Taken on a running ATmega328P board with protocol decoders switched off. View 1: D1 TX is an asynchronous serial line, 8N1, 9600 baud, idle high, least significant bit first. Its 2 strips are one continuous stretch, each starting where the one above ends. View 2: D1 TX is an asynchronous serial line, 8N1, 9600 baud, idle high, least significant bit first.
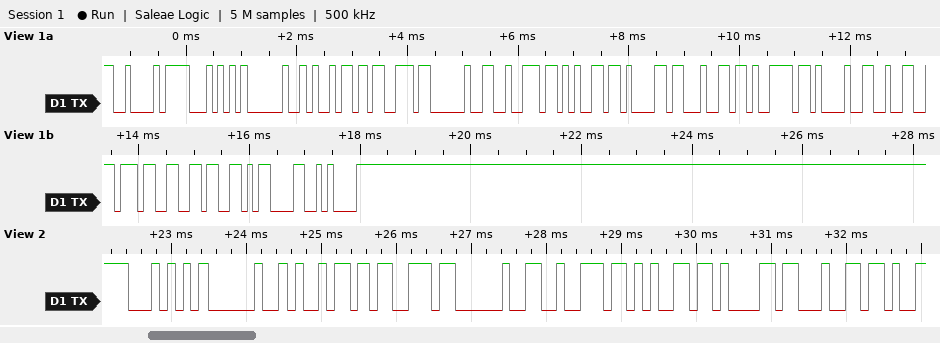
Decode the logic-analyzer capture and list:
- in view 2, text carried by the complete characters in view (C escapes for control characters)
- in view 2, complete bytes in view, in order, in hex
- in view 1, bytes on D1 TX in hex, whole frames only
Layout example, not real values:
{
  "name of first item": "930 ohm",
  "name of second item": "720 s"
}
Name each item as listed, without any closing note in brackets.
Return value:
{
  "in view 2, text carried by the complete characters in view": "\"T is read\"",
  "in view 2, complete bytes in view, in order, in hex": "54 20 69 73 20 72 65 61 64",
  "in view 1, bytes on D1 TX in hex, whole frames only": "0x42 0x54 0x20 0x69 0x73 0x20 0x72 0x65 0x61 0x64 0x79 0x21 0x32 0x37 0x36 0x0D 0x0A"
}
